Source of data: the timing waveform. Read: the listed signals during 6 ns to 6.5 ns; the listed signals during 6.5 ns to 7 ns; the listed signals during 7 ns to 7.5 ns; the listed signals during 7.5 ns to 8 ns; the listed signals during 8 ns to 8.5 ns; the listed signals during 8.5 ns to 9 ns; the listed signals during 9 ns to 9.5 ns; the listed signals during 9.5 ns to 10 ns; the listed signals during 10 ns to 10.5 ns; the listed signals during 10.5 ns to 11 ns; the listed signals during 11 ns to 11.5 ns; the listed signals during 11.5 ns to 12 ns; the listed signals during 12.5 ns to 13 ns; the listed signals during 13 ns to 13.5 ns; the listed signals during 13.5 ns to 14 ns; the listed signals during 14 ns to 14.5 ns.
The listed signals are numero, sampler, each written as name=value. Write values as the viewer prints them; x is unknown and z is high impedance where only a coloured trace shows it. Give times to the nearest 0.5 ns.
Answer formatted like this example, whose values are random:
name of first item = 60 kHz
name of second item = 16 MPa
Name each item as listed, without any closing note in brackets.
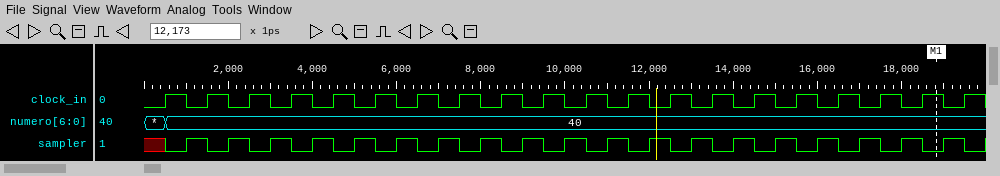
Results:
the listed signals during 6 ns to 6.5 ns = numero=40, sampler=1
the listed signals during 6.5 ns to 7 ns = numero=40, sampler=0
the listed signals during 7 ns to 7.5 ns = numero=40, sampler=1
the listed signals during 7.5 ns to 8 ns = numero=40, sampler=0
the listed signals during 8 ns to 8.5 ns = numero=40, sampler=1
the listed signals during 8.5 ns to 9 ns = numero=40, sampler=0
the listed signals during 9 ns to 9.5 ns = numero=40, sampler=1
the listed signals during 9.5 ns to 10 ns = numero=40, sampler=0
the listed signals during 10 ns to 10.5 ns = numero=40, sampler=1
the listed signals during 10.5 ns to 11 ns = numero=40, sampler=0
the listed signals during 11 ns to 11.5 ns = numero=40, sampler=1
the listed signals during 11.5 ns to 12 ns = numero=40, sampler=0
the listed signals during 12.5 ns to 13 ns = numero=40, sampler=0
the listed signals during 13 ns to 13.5 ns = numero=40, sampler=1
the listed signals during 13.5 ns to 14 ns = numero=40, sampler=0
the listed signals during 14 ns to 14.5 ns = numero=40, sampler=1
